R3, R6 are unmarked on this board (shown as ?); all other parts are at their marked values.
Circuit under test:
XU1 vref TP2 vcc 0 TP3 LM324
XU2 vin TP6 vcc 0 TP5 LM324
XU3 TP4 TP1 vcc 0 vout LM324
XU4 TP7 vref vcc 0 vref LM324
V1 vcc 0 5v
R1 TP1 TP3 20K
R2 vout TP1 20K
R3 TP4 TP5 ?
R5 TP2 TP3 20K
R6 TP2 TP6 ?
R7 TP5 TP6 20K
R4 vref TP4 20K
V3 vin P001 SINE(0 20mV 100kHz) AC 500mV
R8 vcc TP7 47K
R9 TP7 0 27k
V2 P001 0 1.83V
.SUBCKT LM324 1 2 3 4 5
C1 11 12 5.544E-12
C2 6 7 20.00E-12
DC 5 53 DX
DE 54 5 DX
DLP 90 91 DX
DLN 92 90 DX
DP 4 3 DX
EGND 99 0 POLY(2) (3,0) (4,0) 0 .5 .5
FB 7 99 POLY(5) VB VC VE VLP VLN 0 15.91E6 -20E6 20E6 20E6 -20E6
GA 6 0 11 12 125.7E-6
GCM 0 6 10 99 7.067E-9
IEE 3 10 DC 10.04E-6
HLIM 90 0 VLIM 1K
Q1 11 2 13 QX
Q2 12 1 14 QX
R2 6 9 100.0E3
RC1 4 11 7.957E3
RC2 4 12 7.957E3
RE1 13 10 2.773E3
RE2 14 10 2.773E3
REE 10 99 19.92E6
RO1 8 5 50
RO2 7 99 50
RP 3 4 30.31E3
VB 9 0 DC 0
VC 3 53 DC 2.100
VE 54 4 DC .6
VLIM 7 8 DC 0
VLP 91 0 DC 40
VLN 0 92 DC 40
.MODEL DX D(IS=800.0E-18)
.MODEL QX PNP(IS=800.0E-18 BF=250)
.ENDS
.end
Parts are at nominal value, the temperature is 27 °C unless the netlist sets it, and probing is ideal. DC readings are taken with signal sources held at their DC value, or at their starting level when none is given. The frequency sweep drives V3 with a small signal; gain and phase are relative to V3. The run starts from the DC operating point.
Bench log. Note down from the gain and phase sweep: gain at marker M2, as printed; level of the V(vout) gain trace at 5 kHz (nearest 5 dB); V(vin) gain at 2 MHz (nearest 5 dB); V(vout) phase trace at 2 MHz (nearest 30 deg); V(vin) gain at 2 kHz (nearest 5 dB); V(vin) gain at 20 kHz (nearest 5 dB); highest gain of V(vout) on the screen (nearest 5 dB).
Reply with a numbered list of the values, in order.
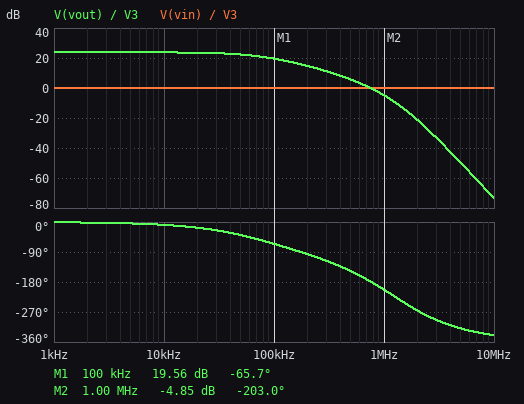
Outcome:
1. -4.85 dB
2. 25 dB
3. 0 dB
4. -270 deg
5. 0 dB
6. 0 dB
7. 25 dB
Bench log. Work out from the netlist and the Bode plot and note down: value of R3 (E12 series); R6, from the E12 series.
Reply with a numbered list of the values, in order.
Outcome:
1. 10 kΩ
2. 3.3 kΩ
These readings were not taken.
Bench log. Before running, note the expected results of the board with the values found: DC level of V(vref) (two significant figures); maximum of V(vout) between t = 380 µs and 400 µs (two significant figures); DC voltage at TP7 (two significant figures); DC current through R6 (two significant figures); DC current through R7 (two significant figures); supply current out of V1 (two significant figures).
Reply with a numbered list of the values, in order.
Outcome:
1. 1.8 V
2. 2.1 V
3. 1.8 V
4. 1.6 µA
5. 1.6 µA
6. 770 µA
